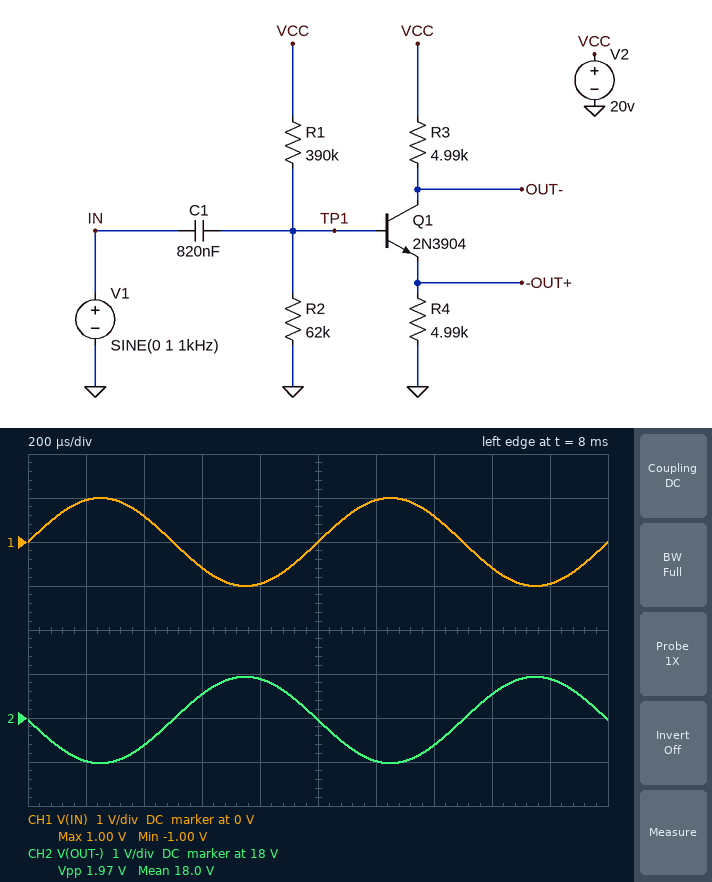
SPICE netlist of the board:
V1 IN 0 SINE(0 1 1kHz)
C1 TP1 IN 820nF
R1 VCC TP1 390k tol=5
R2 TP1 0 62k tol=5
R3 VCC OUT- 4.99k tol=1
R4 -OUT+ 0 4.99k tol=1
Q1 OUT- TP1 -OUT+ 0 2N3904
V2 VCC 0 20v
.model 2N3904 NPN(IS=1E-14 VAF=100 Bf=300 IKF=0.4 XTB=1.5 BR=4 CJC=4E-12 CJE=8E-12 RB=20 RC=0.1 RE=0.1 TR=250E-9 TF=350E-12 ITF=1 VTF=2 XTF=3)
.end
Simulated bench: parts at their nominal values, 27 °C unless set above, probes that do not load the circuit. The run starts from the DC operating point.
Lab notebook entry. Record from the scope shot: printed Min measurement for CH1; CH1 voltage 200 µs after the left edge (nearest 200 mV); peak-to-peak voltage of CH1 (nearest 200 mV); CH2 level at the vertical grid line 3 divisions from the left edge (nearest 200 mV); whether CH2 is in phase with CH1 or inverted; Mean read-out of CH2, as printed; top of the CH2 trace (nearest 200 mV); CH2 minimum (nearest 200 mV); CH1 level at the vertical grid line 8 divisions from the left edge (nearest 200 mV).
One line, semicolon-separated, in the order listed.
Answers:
-1.00 V; 1.0 V; 2.0 V; 18.6 V; inverted; 18.0 V; 19.0 V; 17.0 V; -600 mV
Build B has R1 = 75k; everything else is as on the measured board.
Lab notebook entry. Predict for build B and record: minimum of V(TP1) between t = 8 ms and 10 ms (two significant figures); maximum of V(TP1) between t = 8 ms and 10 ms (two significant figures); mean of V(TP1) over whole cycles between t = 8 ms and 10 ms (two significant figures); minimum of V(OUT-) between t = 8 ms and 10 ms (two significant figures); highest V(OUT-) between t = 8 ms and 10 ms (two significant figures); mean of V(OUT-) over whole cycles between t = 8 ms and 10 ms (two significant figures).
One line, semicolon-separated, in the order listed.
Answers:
7.9 V; 9.9 V; 8.9 V; 11 V; 13 V; 12 V
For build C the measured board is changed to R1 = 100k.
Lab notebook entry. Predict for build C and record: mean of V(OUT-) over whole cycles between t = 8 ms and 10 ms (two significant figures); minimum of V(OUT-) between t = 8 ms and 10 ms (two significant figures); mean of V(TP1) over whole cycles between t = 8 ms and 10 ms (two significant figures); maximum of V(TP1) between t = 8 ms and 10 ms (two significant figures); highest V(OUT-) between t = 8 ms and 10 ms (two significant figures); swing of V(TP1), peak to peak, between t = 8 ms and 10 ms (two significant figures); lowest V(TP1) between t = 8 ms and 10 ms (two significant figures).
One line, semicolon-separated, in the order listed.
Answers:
13 V; 12 V; 7.5 V; 8.5 V; 14 V; 2.0 V; 6.5 V
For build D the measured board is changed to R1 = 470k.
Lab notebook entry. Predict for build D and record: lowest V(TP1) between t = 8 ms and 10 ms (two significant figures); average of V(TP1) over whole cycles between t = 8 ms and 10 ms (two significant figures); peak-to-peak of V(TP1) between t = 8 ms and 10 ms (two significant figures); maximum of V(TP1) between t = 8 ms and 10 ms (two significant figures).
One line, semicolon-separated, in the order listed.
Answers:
1.3 V; 2.3 V; 2.0 V; 3.3 V
